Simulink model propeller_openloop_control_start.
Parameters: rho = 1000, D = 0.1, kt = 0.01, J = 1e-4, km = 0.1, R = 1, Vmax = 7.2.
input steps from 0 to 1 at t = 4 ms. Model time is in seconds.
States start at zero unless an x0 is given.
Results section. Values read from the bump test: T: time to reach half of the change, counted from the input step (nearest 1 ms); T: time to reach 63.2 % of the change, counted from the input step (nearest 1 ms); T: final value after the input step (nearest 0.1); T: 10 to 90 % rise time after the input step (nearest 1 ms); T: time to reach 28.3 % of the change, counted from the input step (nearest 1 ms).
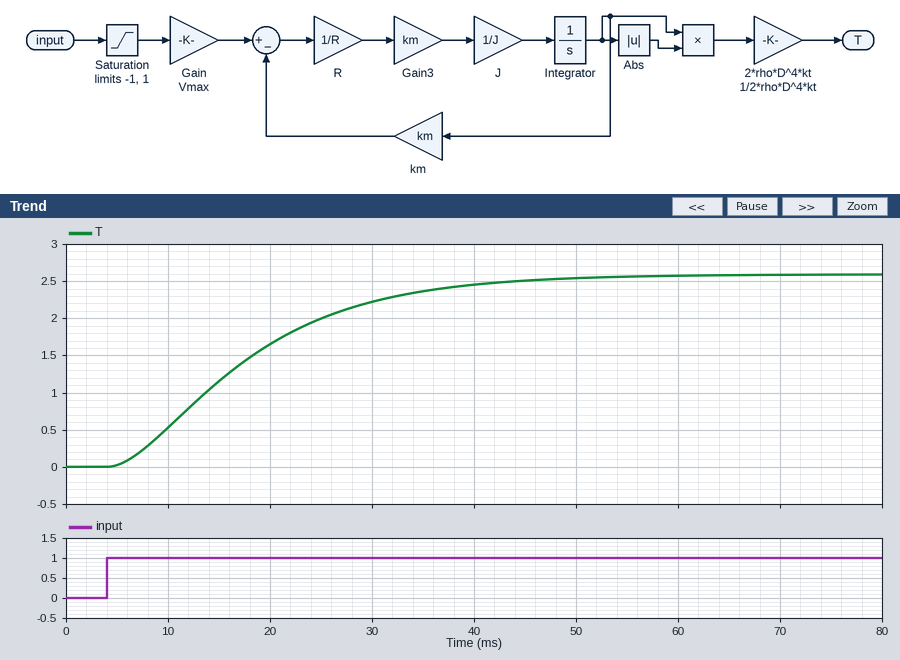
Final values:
12 ms
16 ms
2.6
26 ms
8 ms
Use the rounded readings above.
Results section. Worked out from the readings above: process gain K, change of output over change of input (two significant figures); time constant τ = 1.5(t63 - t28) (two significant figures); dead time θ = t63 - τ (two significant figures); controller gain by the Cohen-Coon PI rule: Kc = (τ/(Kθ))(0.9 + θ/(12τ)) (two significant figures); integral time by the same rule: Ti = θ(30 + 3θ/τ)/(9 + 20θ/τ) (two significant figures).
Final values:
2.6
12 ms
4.0 ms
1.1
7.9 ms
